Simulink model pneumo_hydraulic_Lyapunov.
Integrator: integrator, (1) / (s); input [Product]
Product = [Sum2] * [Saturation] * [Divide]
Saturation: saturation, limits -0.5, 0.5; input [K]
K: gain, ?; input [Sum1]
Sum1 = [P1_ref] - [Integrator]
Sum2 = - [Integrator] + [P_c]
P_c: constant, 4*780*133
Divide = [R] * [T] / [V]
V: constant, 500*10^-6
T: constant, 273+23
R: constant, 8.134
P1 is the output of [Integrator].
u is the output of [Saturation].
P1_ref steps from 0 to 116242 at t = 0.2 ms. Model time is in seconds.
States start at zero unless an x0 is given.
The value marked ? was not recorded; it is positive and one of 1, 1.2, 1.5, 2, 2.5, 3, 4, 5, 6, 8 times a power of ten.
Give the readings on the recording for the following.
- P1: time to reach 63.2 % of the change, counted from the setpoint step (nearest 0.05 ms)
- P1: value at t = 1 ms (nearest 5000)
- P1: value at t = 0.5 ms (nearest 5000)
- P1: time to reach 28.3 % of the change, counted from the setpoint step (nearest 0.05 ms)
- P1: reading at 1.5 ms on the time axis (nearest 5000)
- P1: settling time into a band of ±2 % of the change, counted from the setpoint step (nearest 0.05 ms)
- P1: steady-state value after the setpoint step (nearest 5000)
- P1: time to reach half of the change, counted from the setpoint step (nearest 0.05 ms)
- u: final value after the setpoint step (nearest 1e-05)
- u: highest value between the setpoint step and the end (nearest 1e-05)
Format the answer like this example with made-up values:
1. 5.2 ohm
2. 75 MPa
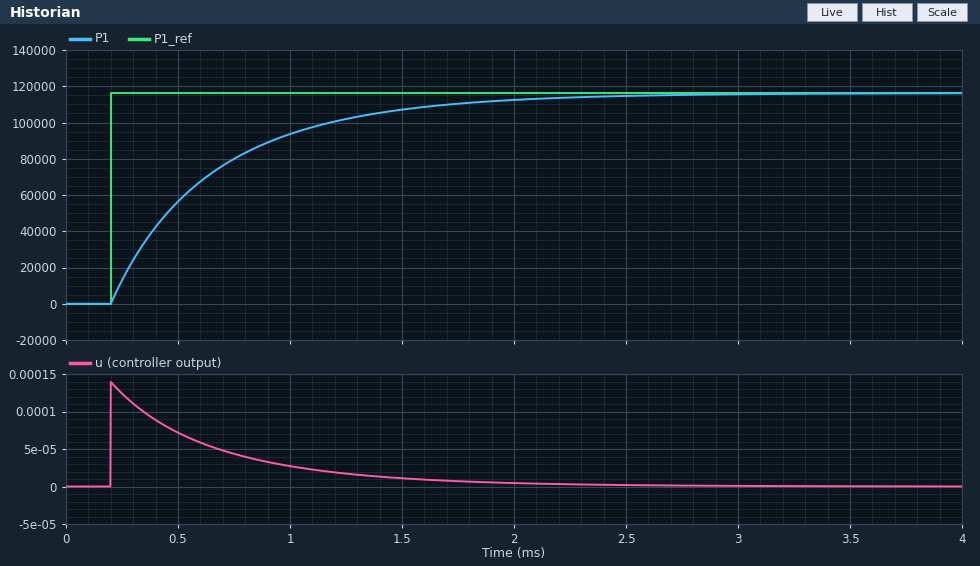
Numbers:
1. 0.45 ms
2. 95000
3. 55000
4. 0.15 ms
5. 105000
6. 2.10 ms
7. 115000
8. 0.30 ms
9. 0.00000
10. 0.00014
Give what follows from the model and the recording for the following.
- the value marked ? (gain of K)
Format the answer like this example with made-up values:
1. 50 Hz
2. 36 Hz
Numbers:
1. 1.2e-09
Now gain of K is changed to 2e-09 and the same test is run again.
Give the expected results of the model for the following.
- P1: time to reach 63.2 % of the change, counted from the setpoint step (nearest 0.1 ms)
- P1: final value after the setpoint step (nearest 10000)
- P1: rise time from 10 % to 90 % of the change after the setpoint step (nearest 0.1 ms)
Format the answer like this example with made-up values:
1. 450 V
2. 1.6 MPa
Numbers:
1. 0.3 ms
2. 120000
3. 0.7 ms
